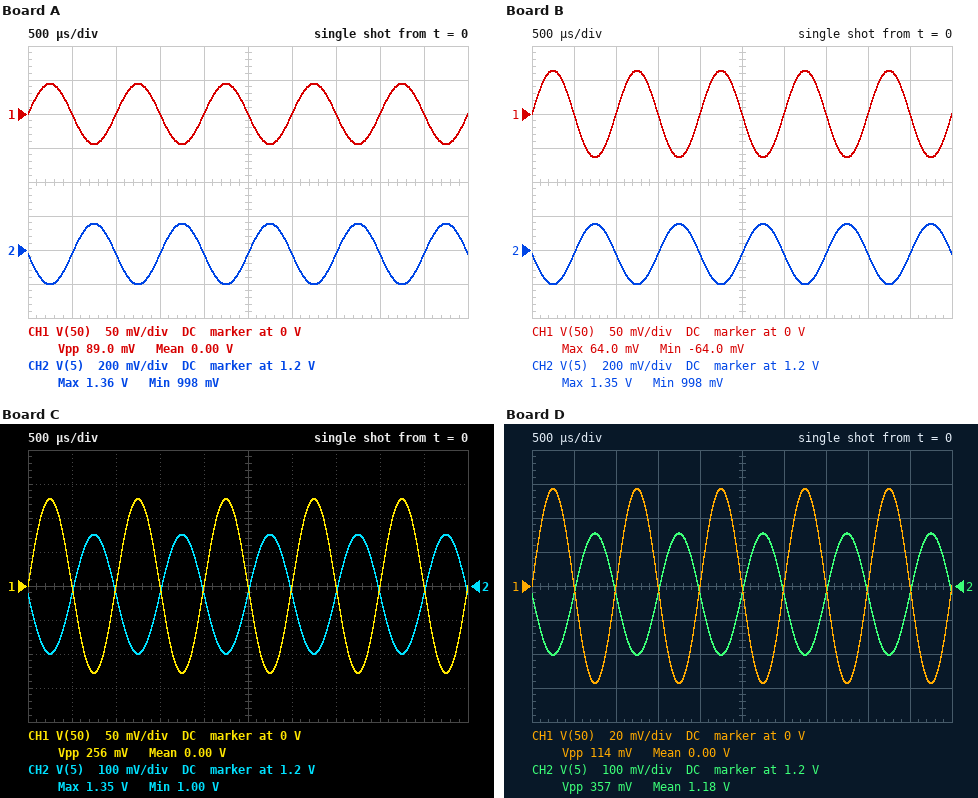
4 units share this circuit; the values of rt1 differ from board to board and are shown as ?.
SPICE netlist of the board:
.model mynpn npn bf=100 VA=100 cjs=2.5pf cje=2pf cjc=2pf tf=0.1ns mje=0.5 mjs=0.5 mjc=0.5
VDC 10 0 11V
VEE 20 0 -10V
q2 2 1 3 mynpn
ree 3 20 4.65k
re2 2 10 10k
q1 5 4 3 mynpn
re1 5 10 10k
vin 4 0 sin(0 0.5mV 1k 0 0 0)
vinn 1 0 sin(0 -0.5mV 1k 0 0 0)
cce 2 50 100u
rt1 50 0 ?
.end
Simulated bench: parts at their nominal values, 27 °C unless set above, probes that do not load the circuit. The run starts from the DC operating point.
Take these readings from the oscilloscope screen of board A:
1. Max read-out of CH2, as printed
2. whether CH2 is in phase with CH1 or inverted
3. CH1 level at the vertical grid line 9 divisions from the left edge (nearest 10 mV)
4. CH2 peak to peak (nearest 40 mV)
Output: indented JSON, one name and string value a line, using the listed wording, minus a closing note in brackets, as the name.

{
  "Max read-out of CH2, as printed": "1.36 V",
  "whether CH2 is in phase with CH1 or inverted": "inverted",
  "CH1 level at the vertical grid line 9 divisions from the left edge": "0 V",
  "CH2 peak to peak": "360 mV"
}
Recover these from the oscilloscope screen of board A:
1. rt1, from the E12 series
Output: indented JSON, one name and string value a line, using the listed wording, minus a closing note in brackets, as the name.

{
  "rt1, from the E12 series": "3.3 kΩ"
}
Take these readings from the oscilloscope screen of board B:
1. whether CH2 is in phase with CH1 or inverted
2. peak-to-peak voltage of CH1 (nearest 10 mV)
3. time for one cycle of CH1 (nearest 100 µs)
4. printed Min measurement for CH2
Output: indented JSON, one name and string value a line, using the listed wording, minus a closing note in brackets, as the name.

{
  "whether CH2 is in phase with CH1 or inverted": "inverted",
  "peak-to-peak voltage of CH1": "130 mV",
  "time for one cycle of CH1": "1.0 ms",
  "printed Min measurement for CH2": "998 mV"
}
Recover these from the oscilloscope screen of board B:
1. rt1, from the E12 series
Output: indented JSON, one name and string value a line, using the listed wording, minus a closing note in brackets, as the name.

{
  "rt1, from the E12 series": "5.6 kΩ"
}
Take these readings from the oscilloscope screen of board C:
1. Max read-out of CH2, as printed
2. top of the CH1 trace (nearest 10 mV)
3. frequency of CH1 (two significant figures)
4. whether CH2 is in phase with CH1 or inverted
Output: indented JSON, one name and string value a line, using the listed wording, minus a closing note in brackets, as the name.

{
  "Max read-out of CH2, as printed": "1.35 V",
  "top of the CH1 trace": "130 mV",
  "frequency of CH1": "1.0 kHz",
  "whether CH2 is in phase with CH1 or inverted": "inverted"
}
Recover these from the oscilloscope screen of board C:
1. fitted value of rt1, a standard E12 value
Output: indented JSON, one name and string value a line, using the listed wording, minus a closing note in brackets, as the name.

{
  "fitted value of rt1, a standard E12 value": "27 kΩ"
}
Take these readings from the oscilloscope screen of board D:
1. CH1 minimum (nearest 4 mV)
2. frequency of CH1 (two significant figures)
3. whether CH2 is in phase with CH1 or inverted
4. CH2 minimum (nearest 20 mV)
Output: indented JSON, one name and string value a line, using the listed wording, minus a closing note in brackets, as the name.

{
  "CH1 minimum": "-56 mV",
  "frequency of CH1": "1.0 kHz",
  "whether CH2 is in phase with CH1 or inverted": "inverted",
  "CH2 minimum": "1.00 V"
}
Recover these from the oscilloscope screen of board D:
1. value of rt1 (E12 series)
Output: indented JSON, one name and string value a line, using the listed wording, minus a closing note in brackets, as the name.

{
  "value of rt1": "4.7 kΩ"
}
